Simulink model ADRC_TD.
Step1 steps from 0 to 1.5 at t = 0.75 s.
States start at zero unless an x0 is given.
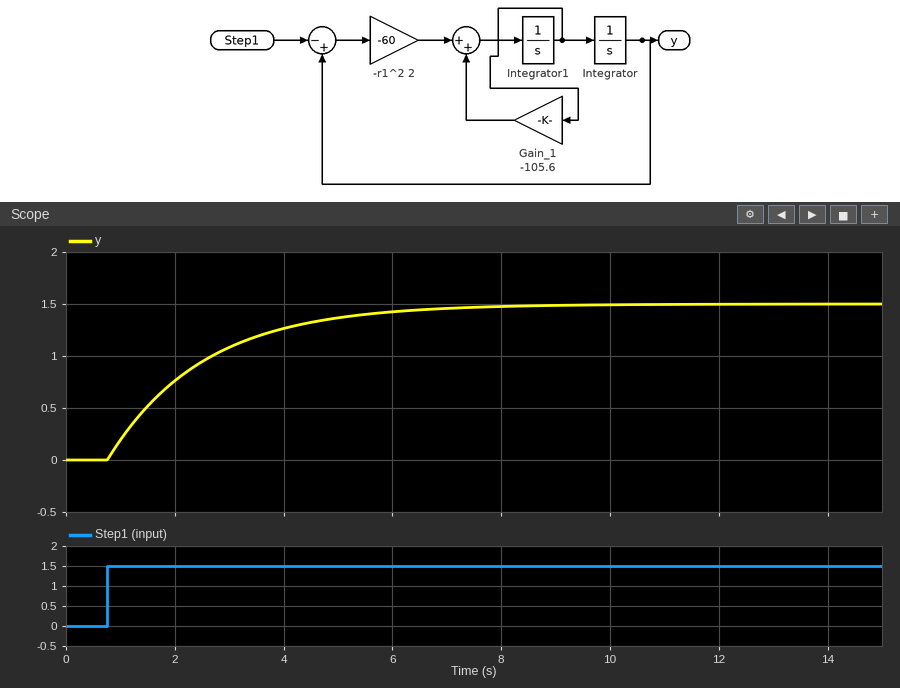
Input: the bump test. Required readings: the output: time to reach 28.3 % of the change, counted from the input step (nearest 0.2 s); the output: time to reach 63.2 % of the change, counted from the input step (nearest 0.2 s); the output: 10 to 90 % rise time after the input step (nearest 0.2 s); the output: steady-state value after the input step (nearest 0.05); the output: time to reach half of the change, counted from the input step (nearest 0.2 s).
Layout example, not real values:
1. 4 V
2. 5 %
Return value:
1. 0.6 s
2. 1.8 s
3. 3.8 s
4. 1.50
5. 1.2 s
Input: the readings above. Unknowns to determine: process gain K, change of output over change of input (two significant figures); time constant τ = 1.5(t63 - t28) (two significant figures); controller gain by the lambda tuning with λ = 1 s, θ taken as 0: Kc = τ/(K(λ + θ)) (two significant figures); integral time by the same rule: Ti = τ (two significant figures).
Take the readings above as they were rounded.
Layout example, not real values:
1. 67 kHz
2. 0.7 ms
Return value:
1. 1.0
2. 1.8 s
3. 1.8
4. 1.8 s
